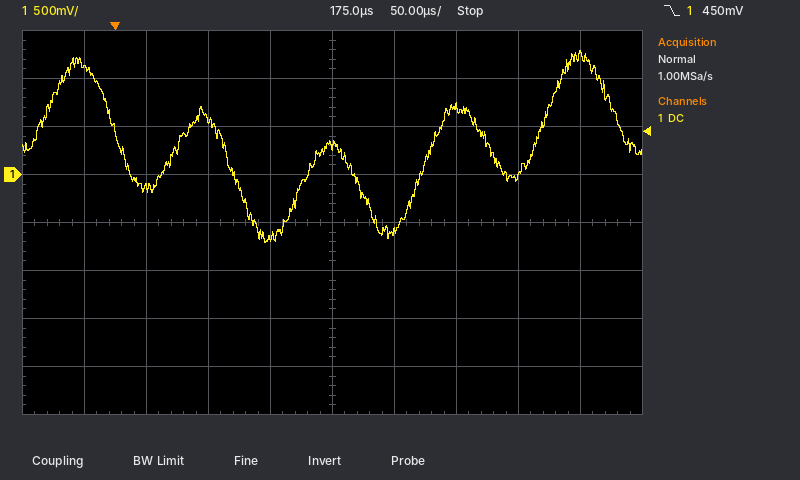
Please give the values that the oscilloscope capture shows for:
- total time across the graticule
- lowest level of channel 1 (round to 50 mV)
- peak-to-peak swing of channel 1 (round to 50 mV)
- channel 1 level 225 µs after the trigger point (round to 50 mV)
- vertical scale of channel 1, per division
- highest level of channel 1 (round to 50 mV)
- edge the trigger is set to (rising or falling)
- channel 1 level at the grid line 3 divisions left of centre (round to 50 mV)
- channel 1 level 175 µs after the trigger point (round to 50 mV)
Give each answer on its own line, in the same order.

500 µs
-700 mV
2.00 V
-600 mV
500 mV
1.30 V
falling
-150 mV
300 mV
